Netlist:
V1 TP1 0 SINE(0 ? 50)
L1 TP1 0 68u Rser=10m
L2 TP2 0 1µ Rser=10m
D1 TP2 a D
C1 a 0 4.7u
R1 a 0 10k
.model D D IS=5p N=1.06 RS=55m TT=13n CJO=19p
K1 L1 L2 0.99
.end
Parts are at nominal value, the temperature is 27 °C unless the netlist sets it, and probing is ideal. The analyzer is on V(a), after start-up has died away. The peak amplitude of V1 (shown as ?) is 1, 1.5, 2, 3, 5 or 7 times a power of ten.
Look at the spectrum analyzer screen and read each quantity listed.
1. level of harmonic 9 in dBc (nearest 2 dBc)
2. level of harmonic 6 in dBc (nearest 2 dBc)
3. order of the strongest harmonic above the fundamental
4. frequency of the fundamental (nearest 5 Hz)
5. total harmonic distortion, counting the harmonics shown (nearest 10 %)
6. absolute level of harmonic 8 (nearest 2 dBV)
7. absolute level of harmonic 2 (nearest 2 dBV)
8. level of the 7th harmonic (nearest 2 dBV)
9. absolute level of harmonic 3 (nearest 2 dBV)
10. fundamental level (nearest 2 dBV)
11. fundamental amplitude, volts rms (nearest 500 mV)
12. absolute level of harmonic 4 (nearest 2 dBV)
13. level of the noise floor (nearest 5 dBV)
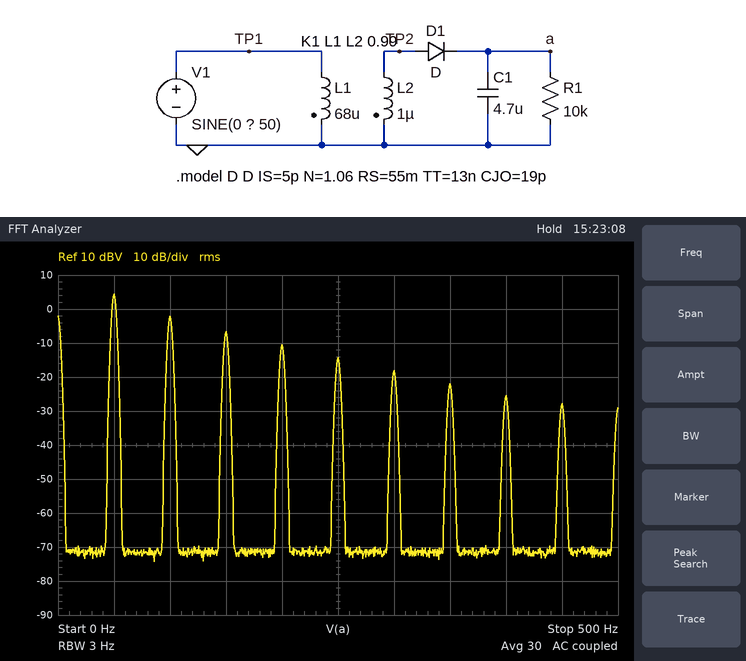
-32 dBc
-22 dBc
2
50 Hz
60 %
-26 dBV
-2 dBV
-22 dBV
-6 dBV
4 dBV
1.5 V
-10 dBV
-70 dBV
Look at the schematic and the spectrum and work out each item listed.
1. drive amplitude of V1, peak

200 V
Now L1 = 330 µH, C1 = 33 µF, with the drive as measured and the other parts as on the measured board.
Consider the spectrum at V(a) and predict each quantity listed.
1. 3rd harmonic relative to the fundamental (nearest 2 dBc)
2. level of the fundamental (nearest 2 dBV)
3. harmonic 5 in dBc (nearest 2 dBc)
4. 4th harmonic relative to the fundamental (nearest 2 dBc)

-10 dBc
-18 dBV
-14 dBc
-12 dBc
